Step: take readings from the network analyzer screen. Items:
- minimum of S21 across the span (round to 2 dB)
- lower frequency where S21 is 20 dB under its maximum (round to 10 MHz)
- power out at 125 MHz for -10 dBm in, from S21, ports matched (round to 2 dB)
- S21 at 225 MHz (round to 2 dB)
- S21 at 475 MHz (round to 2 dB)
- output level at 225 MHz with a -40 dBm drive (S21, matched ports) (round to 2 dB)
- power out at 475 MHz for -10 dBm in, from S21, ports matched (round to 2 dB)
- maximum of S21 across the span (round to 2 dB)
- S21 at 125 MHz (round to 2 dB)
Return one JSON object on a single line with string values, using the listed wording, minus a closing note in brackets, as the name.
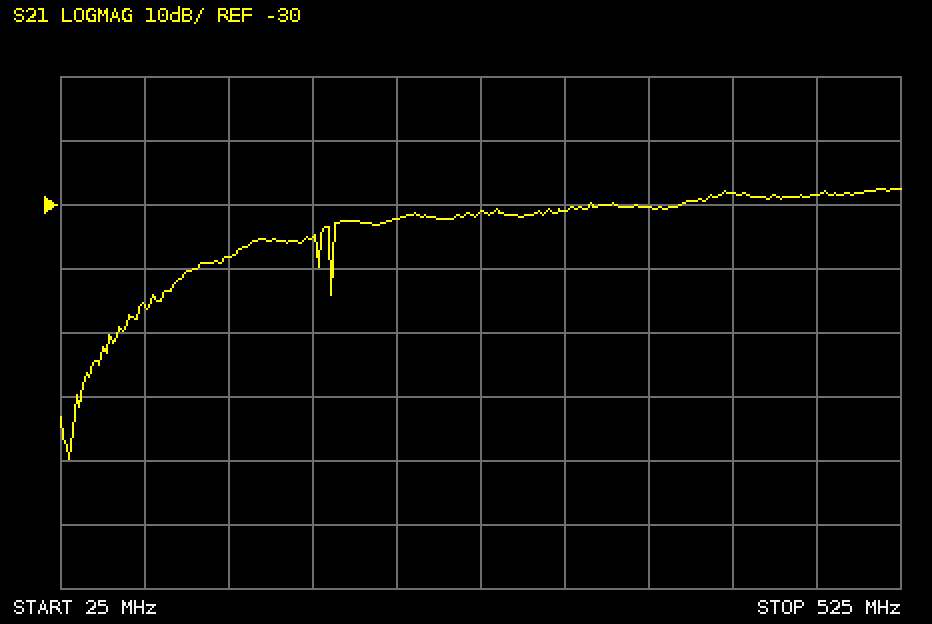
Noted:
{"minimum of S21 across the span": "-70 dB", "lower frequency where S21 is 20 dB under its maximum": "70 MHz", "power out at 125 MHz for -10 dBm in, from S21, ports matched": "-48 dBm", "S21 at 225 MHz": "-32 dB", "S21 at 475 MHz": "-28 dB", "output level at 225 MHz with a -40 dBm drive (S21, matched ports)": "-72 dBm", "power out at 475 MHz for -10 dBm in, from S21, ports matched": "-38 dBm", "maximum of S21 across the span": "-28 dB", "S21 at 125 MHz": "-38 dB"}
